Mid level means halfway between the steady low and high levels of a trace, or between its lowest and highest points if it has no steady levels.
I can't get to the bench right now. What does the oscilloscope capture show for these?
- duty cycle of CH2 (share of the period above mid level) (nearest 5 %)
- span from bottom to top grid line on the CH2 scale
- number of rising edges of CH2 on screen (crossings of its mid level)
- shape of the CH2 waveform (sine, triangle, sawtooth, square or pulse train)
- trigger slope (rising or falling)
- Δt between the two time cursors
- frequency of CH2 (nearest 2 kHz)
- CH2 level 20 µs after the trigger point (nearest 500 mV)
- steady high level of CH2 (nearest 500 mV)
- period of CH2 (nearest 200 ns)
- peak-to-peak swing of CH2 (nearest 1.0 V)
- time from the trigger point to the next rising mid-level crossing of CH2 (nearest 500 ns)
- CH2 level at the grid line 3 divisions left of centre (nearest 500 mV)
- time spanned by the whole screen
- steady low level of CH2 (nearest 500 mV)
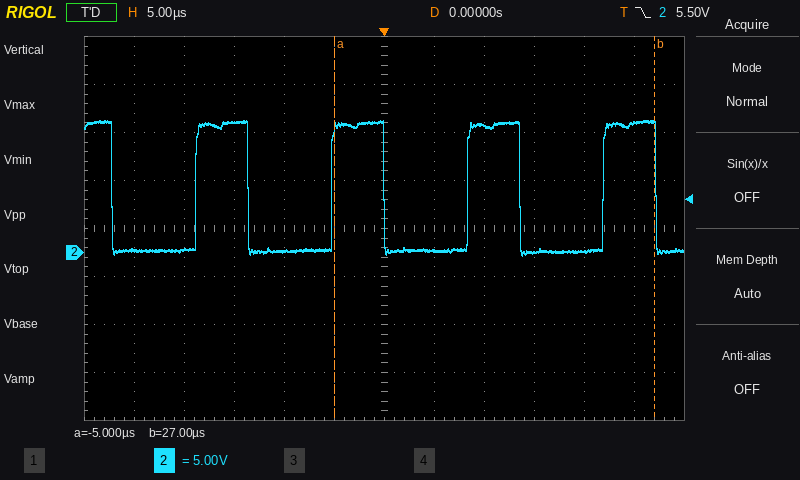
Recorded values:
40 %
40 V
4
pulse train
falling
32.0 µs
74 kHz
0.0 V
13.5 V
13.6 µs
14.0 V
8.5 µs
13.5 V
60 µs
0.0 V
